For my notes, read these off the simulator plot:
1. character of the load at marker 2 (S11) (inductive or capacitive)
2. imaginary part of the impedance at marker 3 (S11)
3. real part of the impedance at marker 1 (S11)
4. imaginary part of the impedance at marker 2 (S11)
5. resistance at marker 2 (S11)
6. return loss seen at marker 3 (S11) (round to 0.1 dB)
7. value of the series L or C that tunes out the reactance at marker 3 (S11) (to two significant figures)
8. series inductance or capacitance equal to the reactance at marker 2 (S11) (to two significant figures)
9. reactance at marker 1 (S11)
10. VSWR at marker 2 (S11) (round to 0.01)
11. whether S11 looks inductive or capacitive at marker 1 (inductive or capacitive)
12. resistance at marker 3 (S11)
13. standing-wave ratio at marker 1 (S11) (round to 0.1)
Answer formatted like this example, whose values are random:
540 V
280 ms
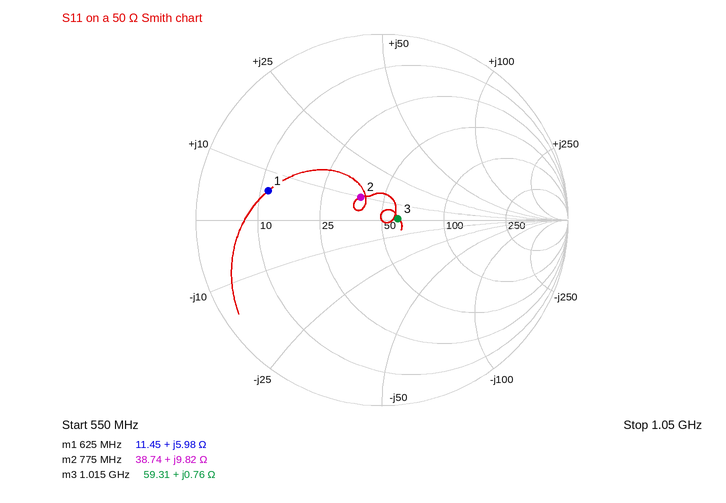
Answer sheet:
inductive
+0.76 Ω
11.45 Ω
+9.82 Ω
38.74 Ω
21.4 dB
210 pF
2.0 nH
+5.98 Ω
1.40
inductive
59.31 Ω
4.4
